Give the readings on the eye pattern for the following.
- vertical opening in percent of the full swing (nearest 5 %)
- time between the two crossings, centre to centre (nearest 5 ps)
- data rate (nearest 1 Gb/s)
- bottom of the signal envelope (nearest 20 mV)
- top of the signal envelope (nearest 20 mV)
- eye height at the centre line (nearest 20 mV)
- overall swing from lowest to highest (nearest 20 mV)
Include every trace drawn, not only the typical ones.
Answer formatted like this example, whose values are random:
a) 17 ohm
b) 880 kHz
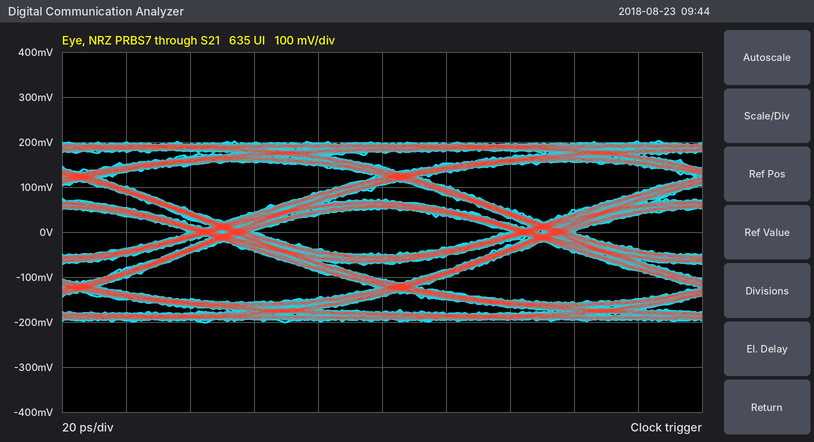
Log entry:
a) 25 %
b) 100 ps
c) 10 Gb/s
d) -200 mV
e) 200 mV
f) 100 mV
g) 400 mV
